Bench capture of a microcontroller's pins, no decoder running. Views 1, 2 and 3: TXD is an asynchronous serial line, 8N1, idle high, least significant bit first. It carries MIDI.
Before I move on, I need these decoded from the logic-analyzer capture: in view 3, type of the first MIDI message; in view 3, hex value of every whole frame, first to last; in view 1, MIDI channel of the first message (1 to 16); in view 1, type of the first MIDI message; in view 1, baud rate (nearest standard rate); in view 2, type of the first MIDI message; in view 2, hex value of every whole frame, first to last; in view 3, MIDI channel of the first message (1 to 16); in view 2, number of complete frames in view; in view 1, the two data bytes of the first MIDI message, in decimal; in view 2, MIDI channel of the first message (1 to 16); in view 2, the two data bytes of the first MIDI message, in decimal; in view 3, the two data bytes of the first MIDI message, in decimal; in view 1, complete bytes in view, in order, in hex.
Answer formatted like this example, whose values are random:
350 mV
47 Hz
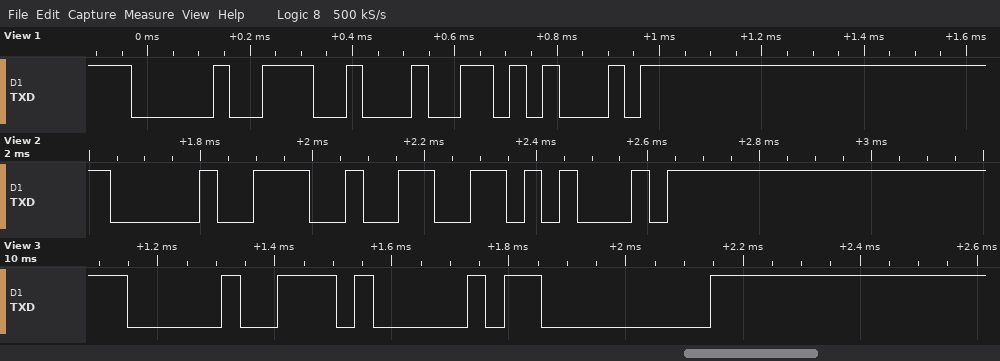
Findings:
Note On
90 41 00
1
Note On
31250 baud
Note On
90 32 45
1
3
34, 69
1
50, 69
65, 0
90 22 45
